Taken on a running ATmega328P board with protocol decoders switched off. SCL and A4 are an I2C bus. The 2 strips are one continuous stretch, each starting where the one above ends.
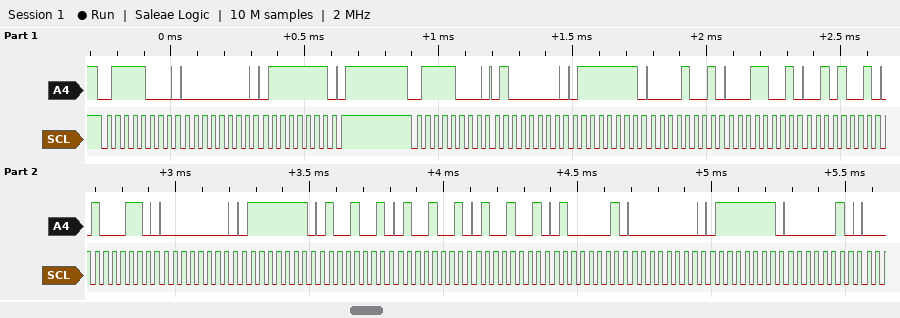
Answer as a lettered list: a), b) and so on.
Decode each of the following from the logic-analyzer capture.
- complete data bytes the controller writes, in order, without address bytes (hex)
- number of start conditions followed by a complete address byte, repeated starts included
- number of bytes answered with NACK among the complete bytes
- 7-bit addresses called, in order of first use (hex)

a) 00 7F 40 7F 09 19 29 46 00 7F 49 49 49 41 00 7F 02
b) 2
c) 0
d) 0x3C
